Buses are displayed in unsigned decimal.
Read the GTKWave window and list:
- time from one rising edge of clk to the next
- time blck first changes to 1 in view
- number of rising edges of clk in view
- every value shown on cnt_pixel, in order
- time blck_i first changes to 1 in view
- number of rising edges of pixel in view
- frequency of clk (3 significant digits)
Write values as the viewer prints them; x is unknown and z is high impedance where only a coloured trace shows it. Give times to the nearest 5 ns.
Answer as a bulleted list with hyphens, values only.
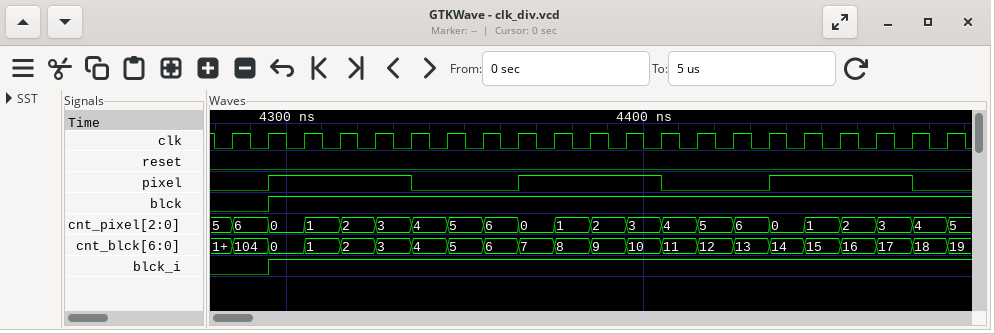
- 10 ns
- 4295 ns
- 21
- 5, 6, 0, 1, 2, 3, 4, 5, 6, 0, 1, 2, 3, 4, 5, 6, 0, 1, 2, 3, 4, 5
- 4295 ns
- 3
- 100 MHz
